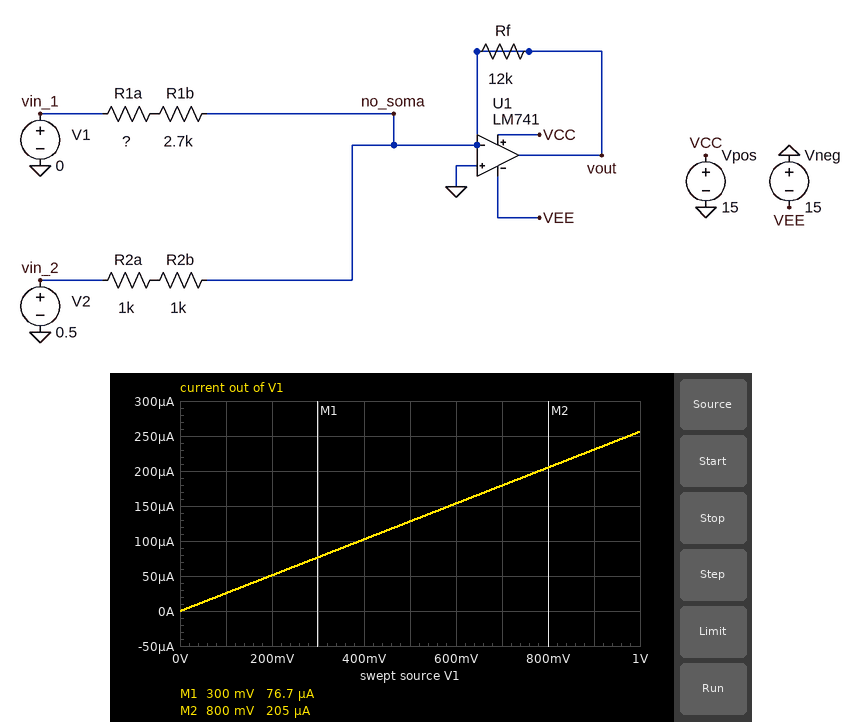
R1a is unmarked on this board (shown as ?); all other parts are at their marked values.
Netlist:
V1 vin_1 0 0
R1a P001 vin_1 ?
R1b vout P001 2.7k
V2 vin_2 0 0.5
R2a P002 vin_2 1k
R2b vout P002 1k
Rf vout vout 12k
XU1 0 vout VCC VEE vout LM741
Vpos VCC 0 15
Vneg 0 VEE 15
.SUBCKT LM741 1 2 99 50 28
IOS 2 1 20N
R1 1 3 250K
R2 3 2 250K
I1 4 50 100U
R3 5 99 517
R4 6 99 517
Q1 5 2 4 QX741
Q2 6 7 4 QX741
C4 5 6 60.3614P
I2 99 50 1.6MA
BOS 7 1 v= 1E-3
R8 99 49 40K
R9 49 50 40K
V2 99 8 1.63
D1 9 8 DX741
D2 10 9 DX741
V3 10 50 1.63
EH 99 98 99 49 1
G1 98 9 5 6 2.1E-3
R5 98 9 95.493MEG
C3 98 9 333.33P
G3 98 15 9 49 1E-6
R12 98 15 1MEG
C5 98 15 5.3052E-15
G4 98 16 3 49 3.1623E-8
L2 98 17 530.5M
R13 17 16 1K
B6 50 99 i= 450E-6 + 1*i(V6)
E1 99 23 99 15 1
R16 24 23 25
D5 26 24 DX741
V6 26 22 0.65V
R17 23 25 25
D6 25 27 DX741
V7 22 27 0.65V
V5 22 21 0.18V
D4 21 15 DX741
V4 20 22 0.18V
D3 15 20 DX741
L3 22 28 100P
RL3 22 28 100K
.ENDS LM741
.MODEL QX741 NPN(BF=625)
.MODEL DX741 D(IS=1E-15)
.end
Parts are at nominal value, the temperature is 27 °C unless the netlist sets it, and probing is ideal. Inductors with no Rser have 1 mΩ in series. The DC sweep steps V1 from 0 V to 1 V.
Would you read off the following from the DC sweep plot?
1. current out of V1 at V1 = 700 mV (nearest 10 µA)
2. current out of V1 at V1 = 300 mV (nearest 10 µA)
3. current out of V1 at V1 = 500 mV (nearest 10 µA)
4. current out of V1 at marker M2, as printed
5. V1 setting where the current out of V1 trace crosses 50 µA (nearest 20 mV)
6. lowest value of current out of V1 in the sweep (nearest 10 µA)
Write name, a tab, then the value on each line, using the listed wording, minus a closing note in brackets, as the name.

current out of V1 at V1 = 700 mV	180 µA
current out of V1 at V1 = 300 mV	80 µA
current out of V1 at V1 = 500 mV	130 µA
current out of V1 at marker M2, as printed	205 µA
V1 setting where the current out of V1 trace crosses 50 µA	200 mV
lowest value of current out of V1 in the sweep	0 A
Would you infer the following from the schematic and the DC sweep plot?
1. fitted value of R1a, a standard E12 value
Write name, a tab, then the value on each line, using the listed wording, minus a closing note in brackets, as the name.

fitted value of R1a, a standard E12 value	1.2 kΩ
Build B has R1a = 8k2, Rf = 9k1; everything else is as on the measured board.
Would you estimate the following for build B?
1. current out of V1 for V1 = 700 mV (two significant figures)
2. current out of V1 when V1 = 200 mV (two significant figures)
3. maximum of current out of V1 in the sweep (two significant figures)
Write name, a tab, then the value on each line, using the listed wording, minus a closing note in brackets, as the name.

current out of V1 for V1 = 700 mV	64 µA
current out of V1 when V1 = 200 mV	18 µA
maximum of current out of V1 in the sweep	92 µA
